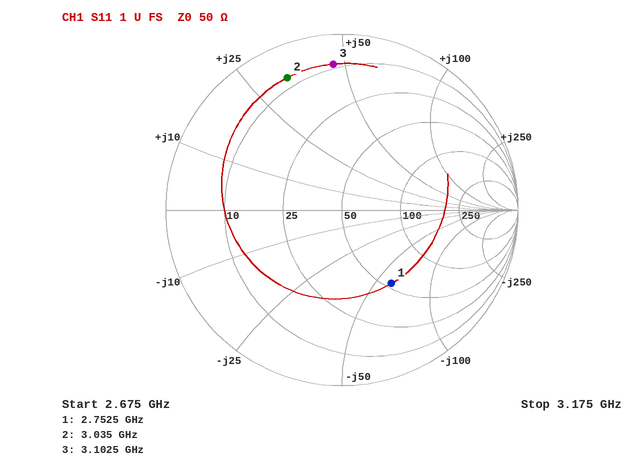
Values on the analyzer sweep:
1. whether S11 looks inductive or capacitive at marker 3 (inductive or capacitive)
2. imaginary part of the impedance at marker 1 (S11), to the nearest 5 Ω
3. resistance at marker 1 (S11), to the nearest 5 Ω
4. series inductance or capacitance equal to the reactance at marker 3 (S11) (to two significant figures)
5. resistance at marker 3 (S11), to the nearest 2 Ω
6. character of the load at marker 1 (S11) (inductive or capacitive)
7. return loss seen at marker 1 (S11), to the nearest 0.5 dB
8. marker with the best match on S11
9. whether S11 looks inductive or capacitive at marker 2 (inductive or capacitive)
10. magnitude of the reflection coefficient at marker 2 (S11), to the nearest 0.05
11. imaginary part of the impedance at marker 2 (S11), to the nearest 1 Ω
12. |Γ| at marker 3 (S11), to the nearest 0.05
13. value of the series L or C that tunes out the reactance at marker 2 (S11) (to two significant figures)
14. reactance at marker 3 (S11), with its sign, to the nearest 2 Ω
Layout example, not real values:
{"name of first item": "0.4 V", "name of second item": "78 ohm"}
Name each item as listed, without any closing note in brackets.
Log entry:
{"whether S11 looks inductive or capacitive at marker 3": "inductive", "imaginary part of the impedance at marker 1 (S11), to the nearest 5 Ω": "-60 Ω", "resistance at marker 1 (S11), to the nearest 5 Ω": "55 Ω", "series inductance or capacitance equal to the reactance at marker 3 (S11)": "2.4 nH", "resistance at marker 3 (S11), to the nearest 2 Ω": "8 Ω", "character of the load at marker 1 (S11)": "capacitive", "return loss seen at marker 1 (S11), to the nearest 0.5 dB": "6.0 dB", "marker with the best match on S11": "marker 1", "whether S11 looks inductive or capacitive at marker 2": "inductive", "magnitude of the reflection coefficient at marker 2 (S11), to the nearest 0.05": "0.80", "imaginary part of the impedance at marker 2 (S11), to the nearest 1 Ω": "+33 Ω", "|Γ| at marker 3 (S11), to the nearest 0.05": "0.85", "value of the series L or C that tunes out the reactance at marker 2 (S11)": "1.6 pF", "reactance at marker 3 (S11), with its sign, to the nearest 2 Ω": "+46 Ω"}
